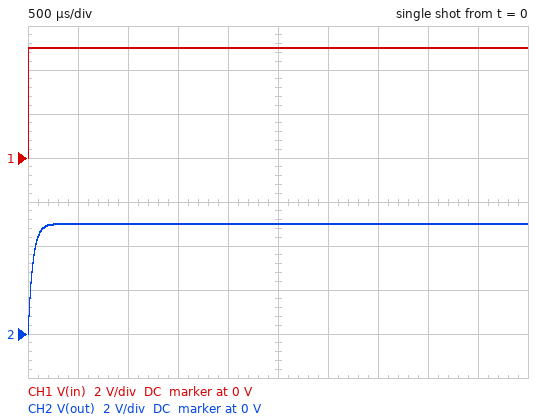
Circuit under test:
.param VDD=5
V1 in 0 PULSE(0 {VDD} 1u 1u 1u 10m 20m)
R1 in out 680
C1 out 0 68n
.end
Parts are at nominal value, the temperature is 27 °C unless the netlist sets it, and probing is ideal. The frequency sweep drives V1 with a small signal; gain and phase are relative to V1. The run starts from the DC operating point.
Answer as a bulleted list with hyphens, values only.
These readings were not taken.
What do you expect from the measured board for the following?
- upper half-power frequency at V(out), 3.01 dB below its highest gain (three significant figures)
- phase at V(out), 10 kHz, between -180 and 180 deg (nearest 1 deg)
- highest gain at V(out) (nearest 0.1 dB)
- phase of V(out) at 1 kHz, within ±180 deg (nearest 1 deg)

- 3.44 kHz
- -71 deg
- 0 dB
- -16 deg
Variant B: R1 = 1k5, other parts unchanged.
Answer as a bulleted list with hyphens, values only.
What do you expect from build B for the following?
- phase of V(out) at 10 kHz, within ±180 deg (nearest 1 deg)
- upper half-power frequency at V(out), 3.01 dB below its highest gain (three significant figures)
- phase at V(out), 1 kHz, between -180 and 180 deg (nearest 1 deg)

- -81 deg
- 1.56 kHz
- -33 deg
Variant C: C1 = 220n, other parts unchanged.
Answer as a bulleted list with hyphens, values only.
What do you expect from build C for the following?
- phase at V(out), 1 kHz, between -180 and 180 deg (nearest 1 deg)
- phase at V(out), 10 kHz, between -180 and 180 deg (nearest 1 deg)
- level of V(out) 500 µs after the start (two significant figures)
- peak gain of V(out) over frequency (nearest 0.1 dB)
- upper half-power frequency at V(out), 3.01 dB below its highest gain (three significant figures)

- -43 deg
- -84 deg
- 4.8 V
- 0 dB
- 1.06 kHz
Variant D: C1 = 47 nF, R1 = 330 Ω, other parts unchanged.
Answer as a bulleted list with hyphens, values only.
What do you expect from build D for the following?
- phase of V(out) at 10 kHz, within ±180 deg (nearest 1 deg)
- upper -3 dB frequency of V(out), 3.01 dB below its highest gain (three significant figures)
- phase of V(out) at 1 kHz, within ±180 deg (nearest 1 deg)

- -44 deg
- 10.3 kHz
- -6 deg
